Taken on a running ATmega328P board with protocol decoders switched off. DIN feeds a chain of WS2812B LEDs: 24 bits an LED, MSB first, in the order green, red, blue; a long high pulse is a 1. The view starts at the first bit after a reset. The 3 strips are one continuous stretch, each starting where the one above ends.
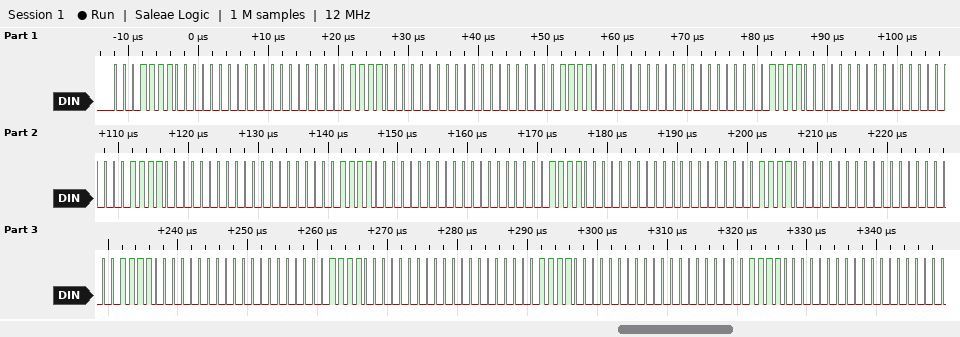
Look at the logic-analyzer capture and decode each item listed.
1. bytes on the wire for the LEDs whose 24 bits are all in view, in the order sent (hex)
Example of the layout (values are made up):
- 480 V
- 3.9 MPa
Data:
- 1E 00 00 1E 00 00 1E 00 00 1E 00 00 1E 00 00 1E 00 00 1E 00 00 1E 00 00 1E 00 00 1E 00 00 1E 00 00 1E 00 00
